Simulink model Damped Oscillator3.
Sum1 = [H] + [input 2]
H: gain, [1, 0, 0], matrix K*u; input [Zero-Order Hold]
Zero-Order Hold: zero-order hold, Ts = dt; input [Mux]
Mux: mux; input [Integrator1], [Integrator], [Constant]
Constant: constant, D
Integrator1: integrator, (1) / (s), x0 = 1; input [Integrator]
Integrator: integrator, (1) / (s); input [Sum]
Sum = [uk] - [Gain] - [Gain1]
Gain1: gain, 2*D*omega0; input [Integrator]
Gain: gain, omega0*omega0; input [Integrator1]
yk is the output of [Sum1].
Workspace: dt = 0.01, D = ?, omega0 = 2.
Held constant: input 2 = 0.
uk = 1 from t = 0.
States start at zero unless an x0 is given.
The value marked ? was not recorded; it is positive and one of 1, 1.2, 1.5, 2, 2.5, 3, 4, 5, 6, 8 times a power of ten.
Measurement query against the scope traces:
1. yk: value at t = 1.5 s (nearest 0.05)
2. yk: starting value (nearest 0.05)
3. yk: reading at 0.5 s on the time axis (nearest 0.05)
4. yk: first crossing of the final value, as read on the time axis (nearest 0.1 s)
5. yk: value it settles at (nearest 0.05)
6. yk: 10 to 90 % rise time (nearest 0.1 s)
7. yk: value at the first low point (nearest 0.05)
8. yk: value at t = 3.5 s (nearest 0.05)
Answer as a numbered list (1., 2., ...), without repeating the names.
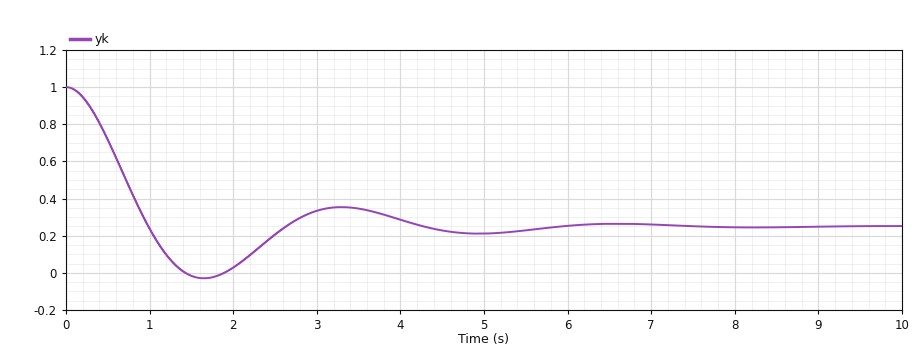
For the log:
1. 0.00
2. 1.00
3. 0.70
4. 1.0 s
5. 0.25
6. 0.7 s
7. -0.05
8. 0.35
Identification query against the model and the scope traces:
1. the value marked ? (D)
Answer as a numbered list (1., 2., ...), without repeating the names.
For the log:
1. 0.3
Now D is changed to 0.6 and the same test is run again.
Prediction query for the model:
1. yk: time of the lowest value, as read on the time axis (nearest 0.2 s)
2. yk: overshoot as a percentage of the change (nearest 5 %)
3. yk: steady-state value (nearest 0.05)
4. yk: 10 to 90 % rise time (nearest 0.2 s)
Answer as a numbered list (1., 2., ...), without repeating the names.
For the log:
1. 2.0 s
2. 10 %
3. 0.25
4. 1.0 s
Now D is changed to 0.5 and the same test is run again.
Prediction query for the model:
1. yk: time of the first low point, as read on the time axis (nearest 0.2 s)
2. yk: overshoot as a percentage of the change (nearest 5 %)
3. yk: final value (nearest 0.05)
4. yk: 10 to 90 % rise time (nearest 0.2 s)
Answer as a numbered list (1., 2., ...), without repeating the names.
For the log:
1. 1.8 s
2. 15 %
3. 0.25
4. 0.8 s
